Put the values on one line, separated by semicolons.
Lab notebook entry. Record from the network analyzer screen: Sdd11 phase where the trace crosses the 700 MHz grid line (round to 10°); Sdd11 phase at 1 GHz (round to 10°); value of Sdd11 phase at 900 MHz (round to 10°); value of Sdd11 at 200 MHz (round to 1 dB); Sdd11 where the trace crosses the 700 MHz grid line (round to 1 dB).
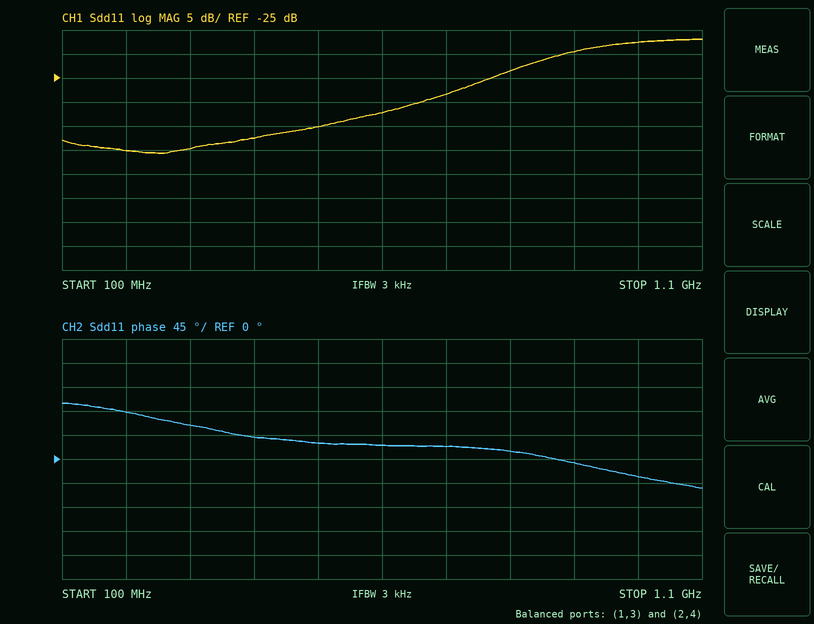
20°; -30°; -10°; -40 dB; -28 dB
